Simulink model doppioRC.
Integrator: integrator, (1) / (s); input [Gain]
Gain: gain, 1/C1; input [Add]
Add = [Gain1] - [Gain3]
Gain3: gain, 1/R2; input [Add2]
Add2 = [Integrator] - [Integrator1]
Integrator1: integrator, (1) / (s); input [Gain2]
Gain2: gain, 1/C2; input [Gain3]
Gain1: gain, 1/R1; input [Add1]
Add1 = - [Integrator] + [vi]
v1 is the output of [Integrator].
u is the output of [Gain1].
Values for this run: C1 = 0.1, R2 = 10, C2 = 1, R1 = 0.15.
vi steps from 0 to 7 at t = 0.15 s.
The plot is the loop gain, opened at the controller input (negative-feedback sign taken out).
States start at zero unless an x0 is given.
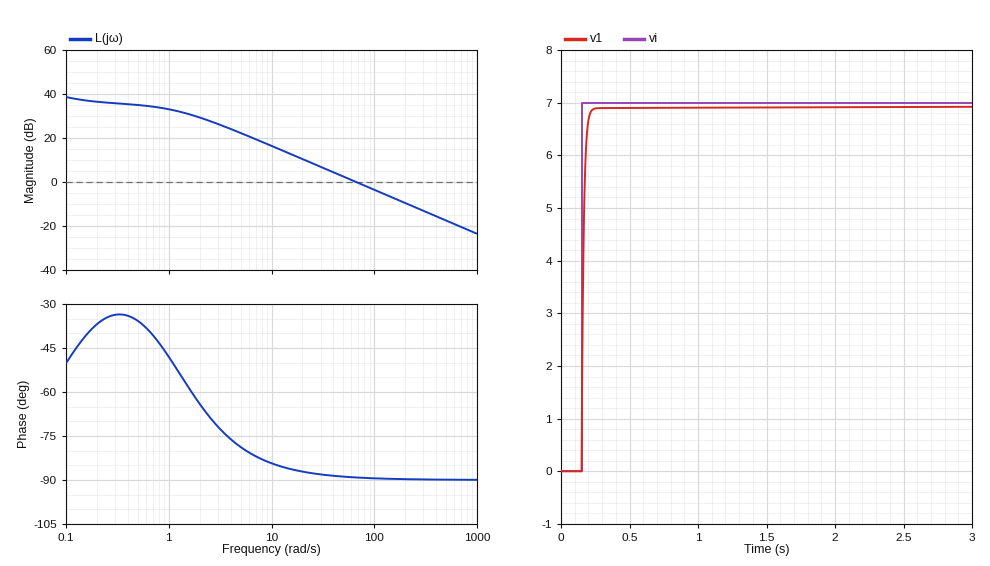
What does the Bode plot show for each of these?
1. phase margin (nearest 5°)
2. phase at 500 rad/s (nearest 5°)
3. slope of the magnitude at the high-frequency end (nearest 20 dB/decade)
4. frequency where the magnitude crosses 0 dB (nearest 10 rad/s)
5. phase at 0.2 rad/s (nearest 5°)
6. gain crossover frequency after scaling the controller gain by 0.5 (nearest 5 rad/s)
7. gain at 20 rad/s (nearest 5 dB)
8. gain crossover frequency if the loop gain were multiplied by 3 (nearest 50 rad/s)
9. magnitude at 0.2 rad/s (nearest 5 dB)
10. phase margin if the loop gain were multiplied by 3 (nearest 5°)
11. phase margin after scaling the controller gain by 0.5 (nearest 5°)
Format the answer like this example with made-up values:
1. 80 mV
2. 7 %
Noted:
1. 90°
2. -90°
3. -20 dB/decade
4. 70 rad/s
5. -35°
6. 35 rad/s
7. 10 dB
8. 200 rad/s
9. 35 dB
10. 90°
11. 90°
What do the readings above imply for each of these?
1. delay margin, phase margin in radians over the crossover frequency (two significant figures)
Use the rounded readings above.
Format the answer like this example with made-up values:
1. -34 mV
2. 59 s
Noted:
1. 0.022 s
